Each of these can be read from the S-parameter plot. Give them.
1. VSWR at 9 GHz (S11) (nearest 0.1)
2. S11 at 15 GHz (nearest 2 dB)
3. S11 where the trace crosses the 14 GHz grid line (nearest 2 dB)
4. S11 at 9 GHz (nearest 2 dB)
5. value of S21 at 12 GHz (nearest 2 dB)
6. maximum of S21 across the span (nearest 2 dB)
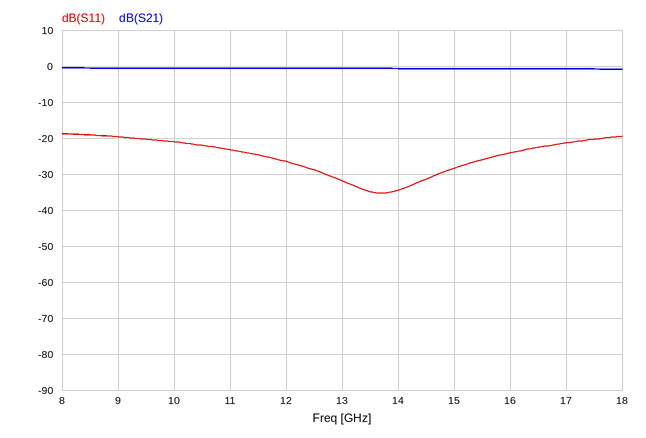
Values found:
1.2
-28 dB
-34 dB
-20 dB
0 dB
0 dB
